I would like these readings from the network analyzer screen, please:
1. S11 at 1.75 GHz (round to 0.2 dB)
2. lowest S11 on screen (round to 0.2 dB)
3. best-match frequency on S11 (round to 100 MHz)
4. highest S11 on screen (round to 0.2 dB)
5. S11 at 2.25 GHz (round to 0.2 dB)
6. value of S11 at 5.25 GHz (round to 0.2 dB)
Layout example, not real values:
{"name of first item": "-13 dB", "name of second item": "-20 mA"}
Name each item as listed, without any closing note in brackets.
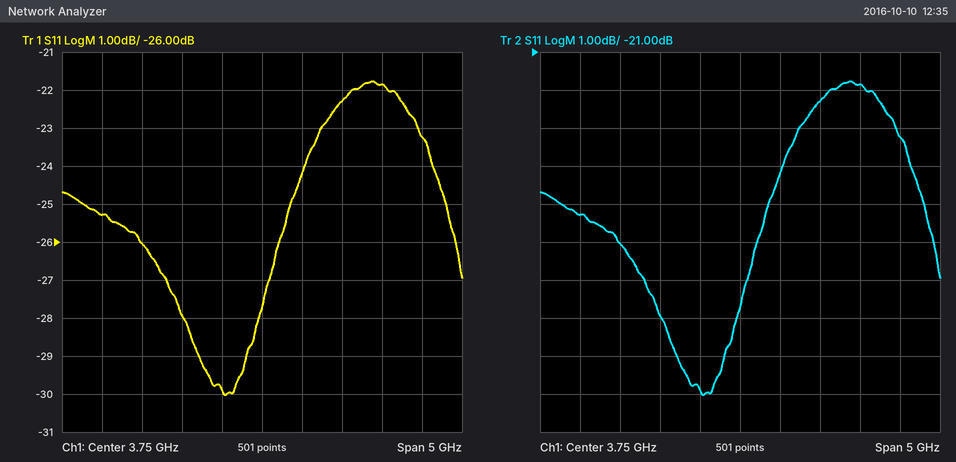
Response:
{"S11 at 1.75 GHz": "-25.2 dB", "lowest S11 on screen": "-30.0 dB", "best-match frequency on S11": "3.3 GHz", "highest S11 on screen": "-21.8 dB", "S11 at 2.25 GHz": "-26.0 dB", "value of S11 at 5.25 GHz": "-21.8 dB"}
